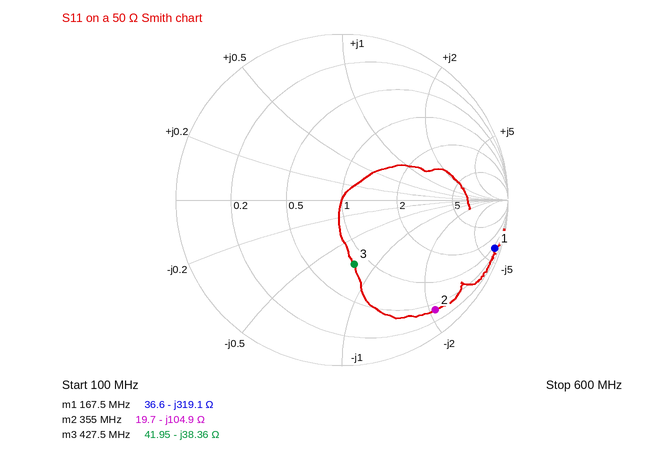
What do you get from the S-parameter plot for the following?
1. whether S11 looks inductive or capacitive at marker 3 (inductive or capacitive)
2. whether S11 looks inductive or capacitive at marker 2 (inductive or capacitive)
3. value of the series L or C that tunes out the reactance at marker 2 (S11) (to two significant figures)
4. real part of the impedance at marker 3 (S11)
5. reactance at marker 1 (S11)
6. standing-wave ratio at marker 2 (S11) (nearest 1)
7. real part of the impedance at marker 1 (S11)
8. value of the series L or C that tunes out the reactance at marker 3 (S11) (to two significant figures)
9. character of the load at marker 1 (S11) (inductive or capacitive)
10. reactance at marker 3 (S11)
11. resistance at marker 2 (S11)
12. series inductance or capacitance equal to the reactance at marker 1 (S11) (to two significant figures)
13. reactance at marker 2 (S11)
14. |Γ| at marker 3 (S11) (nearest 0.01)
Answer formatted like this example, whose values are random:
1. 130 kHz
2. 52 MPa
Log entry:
1. capacitive
2. capacitive
3. 47 nH
4. 41.95 Ω
5. -319.1 Ω
6. 14
7. 36.6 Ω
8. 14 nH
9. capacitive
10. -38.36 Ω
11. 19.7 Ω
12. 3.0 pF
13. -104.9 Ω
14. 0.39
